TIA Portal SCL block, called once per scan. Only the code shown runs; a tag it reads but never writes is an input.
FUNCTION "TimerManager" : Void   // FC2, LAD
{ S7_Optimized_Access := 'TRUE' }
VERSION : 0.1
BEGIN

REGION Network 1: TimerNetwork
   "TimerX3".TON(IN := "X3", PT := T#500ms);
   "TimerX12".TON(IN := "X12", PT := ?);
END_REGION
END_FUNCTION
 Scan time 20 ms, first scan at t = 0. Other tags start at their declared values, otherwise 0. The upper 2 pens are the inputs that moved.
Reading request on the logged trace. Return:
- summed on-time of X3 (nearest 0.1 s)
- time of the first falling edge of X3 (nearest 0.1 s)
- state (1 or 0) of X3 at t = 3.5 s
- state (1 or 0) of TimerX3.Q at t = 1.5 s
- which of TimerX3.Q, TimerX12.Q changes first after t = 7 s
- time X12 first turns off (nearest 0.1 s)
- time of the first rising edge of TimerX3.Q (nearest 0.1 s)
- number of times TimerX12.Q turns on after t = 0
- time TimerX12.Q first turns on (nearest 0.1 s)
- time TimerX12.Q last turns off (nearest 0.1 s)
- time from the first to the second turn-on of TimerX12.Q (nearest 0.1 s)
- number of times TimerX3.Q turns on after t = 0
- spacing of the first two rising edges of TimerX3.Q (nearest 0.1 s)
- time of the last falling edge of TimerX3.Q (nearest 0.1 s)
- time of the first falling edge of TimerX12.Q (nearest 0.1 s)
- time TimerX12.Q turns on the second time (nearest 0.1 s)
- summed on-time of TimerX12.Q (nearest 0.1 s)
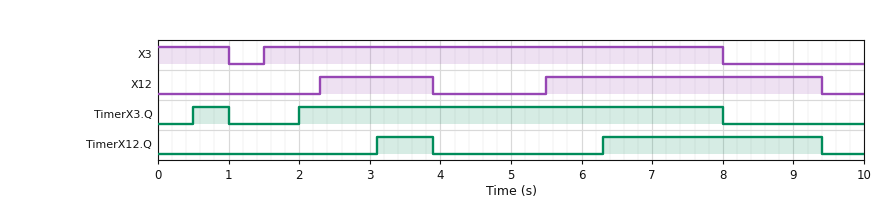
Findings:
7.5 s
1.0 s
1
0
TimerX3.Q
3.9 s
0.5 s
2
3.1 s
9.4 s
3.2 s
2
1.5 s
8.0 s
3.9 s
6.3 s
3.9 s
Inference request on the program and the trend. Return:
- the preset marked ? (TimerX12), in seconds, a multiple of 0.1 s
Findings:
0.8 s
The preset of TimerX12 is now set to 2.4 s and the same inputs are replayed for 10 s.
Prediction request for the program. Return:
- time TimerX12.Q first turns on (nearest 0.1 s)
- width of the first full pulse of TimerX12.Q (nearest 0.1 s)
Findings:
7.9 s
1.5 s
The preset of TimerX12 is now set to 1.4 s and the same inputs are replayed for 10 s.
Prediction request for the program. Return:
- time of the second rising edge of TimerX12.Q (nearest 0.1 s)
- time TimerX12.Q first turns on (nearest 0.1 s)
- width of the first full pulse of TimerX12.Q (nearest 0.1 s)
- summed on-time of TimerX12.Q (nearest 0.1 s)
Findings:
6.9 s
3.7 s
0.2 s
2.7 s
